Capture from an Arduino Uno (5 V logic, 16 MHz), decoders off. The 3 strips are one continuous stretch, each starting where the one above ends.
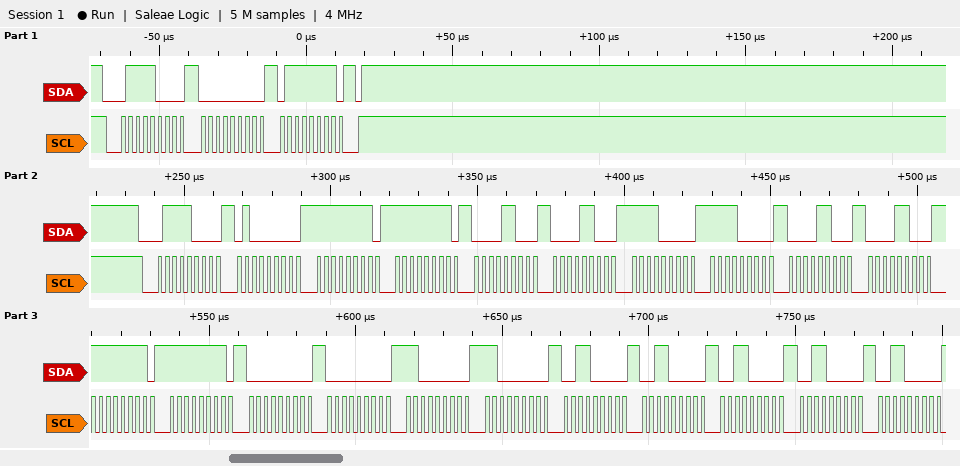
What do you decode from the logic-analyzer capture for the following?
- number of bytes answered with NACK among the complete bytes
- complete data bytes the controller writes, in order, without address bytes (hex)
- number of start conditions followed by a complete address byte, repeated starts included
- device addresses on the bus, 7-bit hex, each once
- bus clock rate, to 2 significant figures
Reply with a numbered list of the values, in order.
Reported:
1. 0
2. 00 7F 40 FF FF 0C 0C F0 F0 0C 0C FF FF 00 00 C0 C0 30 30 30 30 30
3. 2
4. 0x3C
5. 400 kHz
